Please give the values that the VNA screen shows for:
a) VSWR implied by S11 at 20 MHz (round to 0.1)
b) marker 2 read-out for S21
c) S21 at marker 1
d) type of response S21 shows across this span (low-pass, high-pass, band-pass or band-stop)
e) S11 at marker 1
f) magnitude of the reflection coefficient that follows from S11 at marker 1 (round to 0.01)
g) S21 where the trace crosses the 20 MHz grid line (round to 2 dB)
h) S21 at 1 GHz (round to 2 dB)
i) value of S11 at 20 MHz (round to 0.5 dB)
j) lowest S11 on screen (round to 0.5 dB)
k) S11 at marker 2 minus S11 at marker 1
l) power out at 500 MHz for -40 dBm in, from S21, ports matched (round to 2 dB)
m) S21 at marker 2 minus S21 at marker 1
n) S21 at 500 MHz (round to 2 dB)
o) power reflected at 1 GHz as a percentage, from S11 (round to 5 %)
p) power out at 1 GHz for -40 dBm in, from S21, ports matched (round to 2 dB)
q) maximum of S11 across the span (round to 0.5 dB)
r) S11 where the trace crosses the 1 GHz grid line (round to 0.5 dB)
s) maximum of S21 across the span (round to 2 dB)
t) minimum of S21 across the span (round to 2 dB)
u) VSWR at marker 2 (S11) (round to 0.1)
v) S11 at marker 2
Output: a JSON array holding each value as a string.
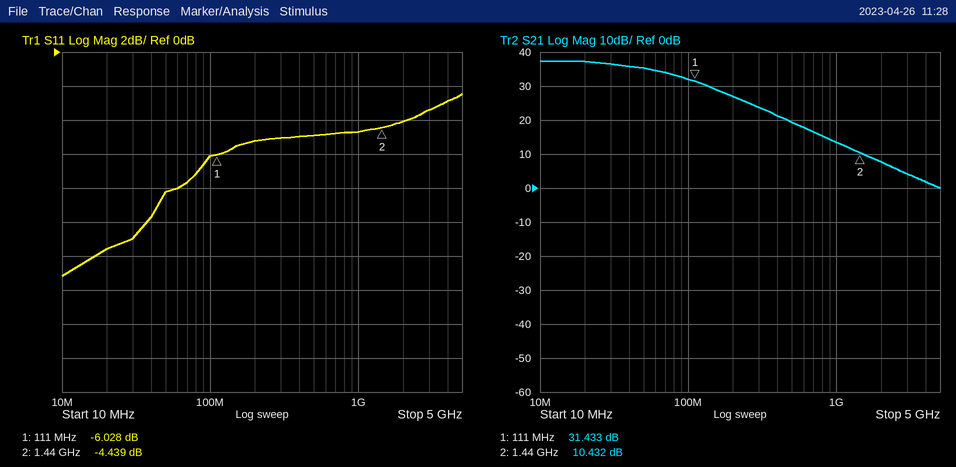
["1.7", "10.432 dB", "31.433 dB", "low-pass", "-6.028 dB", "0.50", "38 dB", "14 dB", "-11.5 dB", "-13.0 dB", "1.589 dB", "-20 dBm", "-21.001 dB", "20 dB", "35 %", "-26 dBm", "-2.5 dB", "-4.5 dB", "38 dB", "0 dB", "4.0", "-4.439 dB"]
